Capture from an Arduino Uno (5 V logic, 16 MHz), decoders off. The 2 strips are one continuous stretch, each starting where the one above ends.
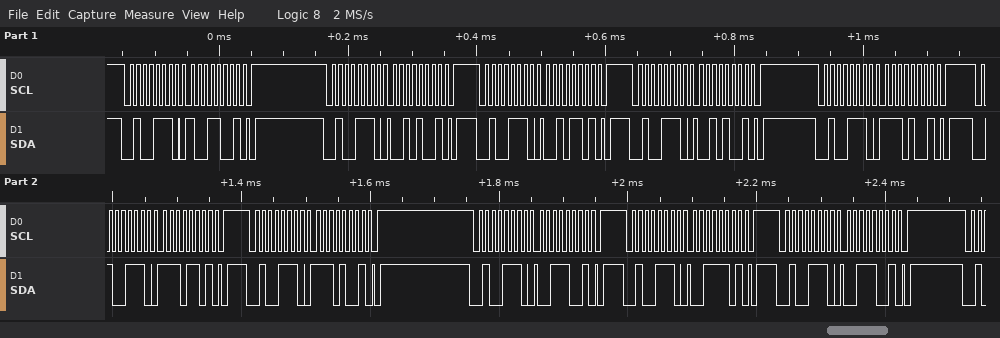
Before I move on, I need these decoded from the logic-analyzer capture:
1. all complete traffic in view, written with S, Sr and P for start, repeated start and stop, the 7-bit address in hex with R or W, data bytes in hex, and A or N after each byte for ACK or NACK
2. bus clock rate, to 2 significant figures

S 27W A 99 A P S 27W A 29 A P S 27W A 2D A P S 27W A 29 A P S 27W A E9 A P S 27W A ED A P S 27W A E9 A P S 27W A 39 A P S 27W A 3D A P S 27W A 39 A P
100 kHz
